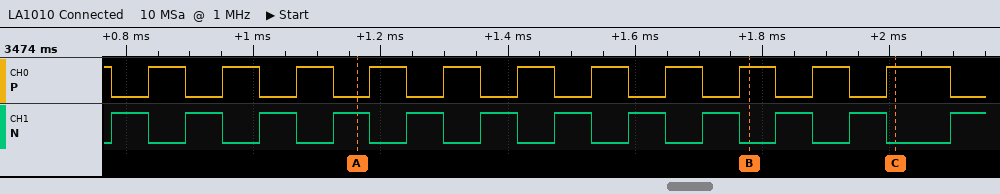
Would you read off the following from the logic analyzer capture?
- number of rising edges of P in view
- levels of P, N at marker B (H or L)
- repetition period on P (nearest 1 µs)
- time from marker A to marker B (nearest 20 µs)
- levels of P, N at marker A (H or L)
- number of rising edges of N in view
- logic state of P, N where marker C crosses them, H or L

11
P=H, N=L
116 µs
620 µs
P=L, N=H
12
P=H, N=L
